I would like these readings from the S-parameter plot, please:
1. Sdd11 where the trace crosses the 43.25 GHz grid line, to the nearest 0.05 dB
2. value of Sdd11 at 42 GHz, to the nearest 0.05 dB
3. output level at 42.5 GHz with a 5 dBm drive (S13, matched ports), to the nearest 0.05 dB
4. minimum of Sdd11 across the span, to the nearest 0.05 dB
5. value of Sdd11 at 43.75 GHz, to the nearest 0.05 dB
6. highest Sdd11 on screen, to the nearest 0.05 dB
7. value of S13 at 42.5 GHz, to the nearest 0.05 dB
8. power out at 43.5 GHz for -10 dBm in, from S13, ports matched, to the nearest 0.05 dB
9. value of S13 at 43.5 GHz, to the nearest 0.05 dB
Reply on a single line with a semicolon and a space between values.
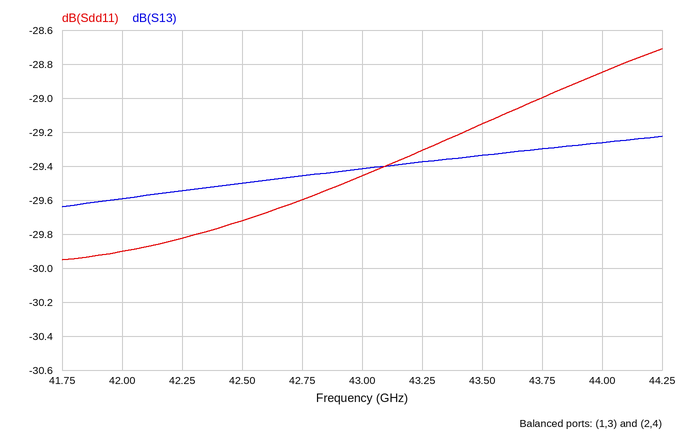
-29.30 dB; -29.90 dB; -24.50 dBm; -29.95 dB; -29.00 dB; -28.70 dB; -29.50 dB; -39.35 dBm; -29.35 dB
